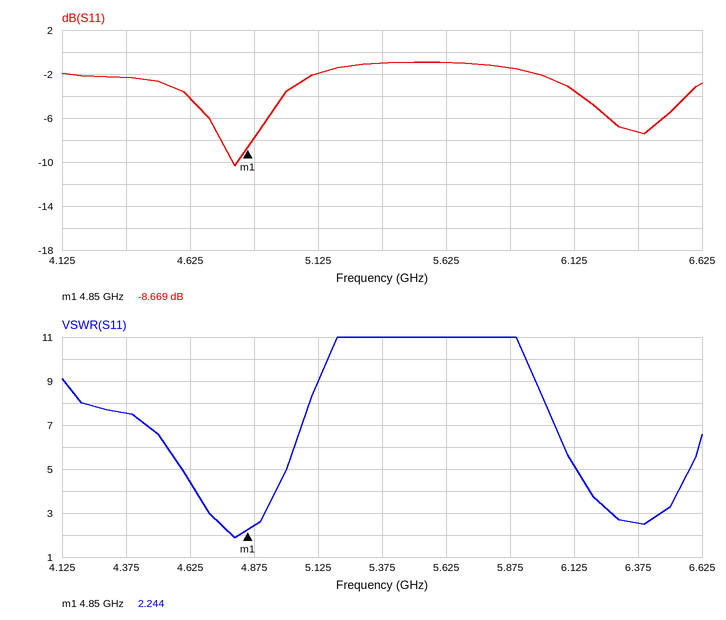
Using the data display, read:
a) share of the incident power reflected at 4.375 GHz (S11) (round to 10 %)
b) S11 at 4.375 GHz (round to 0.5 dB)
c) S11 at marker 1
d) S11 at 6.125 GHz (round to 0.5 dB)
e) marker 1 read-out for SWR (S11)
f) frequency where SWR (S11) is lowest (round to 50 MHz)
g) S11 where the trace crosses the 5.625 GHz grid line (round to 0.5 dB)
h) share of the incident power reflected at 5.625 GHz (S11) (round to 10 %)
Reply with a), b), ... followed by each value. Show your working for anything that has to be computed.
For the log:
a) 10^(-2.5/10) ≈ 56.2 %, so 60 % to the nearest 10 %
b) -2.5 dB
c) -8.669 dB
d) -3.5 dB
e) 2.244
f) 4.80 GHz
g) -1.0 dB
h) 10^(-1/10) ≈ 79.4 %, so 80 % to the nearest 10 %
